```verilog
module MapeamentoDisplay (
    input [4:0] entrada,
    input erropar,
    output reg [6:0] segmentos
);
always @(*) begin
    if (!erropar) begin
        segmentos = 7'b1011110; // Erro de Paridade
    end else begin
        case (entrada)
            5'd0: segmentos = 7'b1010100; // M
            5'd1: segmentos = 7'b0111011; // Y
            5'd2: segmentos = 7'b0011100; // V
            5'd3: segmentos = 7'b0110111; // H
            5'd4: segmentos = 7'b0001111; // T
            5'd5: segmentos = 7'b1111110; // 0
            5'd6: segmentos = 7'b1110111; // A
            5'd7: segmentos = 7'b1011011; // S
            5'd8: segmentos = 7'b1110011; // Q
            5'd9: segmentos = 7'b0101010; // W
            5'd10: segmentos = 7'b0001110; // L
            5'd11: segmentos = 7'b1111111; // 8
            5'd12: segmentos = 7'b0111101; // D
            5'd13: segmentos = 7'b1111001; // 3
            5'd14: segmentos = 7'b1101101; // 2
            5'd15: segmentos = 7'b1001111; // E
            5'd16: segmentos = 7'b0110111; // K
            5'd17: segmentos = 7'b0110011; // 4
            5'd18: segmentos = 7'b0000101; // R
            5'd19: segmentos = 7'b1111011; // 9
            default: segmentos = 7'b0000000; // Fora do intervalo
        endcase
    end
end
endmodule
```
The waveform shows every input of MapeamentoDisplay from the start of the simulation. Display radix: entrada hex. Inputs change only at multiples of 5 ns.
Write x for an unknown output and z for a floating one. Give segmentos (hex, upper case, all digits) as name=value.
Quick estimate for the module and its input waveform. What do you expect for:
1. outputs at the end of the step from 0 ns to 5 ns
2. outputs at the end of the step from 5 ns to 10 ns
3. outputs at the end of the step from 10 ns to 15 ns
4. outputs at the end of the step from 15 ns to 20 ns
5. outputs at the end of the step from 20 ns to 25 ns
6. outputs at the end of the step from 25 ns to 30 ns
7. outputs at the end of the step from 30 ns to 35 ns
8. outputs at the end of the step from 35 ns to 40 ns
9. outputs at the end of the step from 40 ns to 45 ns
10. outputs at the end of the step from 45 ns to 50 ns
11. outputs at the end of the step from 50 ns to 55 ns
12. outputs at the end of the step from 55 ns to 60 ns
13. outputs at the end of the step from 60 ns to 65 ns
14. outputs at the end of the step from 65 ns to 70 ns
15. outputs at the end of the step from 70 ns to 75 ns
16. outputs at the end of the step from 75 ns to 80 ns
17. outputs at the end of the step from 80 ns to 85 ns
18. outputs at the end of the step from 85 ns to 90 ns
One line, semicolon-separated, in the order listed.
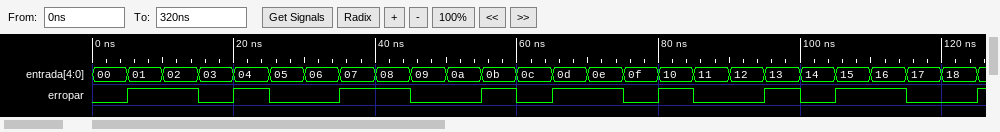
segmentos=5E; segmentos=3B; segmentos=1C; segmentos=5E; segmentos=0F; segmentos=5E; segmentos=5E; segmentos=5B; segmentos=73; segmentos=5E; segmentos=5E; segmentos=7F; segmentos=5E; segmentos=79; segmentos=6D; segmentos=5E; segmentos=37; segmentos=5E
